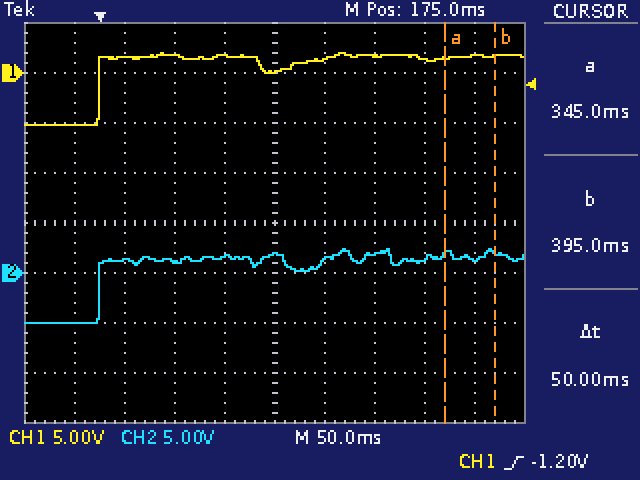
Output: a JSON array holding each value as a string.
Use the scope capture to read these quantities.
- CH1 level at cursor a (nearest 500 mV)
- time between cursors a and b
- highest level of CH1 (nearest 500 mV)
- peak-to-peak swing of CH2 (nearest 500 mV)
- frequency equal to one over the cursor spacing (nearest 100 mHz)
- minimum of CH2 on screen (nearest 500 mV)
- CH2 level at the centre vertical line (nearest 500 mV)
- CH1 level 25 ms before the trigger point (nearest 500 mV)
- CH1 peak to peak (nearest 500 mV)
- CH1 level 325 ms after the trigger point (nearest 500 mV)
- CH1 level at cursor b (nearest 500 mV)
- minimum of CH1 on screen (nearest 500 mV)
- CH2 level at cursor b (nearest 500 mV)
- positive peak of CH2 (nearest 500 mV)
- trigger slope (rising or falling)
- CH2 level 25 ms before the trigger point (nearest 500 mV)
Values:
["1.5 V", "50 ms", "2.0 V", "7.5 V", "20.0 Hz", "-5.0 V", "2.0 V", "-5.0 V", "7.0 V", "1.5 V", "1.5 V", "-5.0 V", "2.0 V", "2.5 V", "rising", "-5.0 V"]
